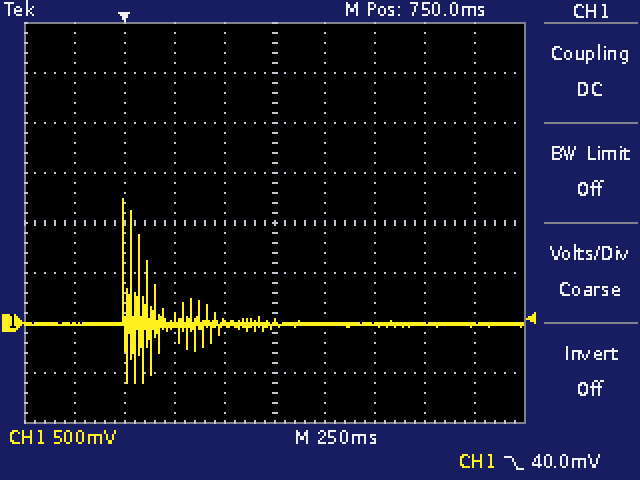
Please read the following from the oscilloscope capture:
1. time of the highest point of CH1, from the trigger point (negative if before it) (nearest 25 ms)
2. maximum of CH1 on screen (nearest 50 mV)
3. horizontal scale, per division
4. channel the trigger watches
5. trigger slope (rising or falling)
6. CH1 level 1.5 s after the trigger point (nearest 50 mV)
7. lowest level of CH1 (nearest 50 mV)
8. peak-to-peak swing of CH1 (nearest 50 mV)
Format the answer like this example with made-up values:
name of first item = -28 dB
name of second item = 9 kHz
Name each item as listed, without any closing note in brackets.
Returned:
time of the highest point of CH1, from the trigger point (negative if before it) = 0 ms
maximum of CH1 on screen = 1.25 V
horizontal scale, per division = 250 ms
channel the trigger watches = CH1
trigger slope = falling
CH1 level 1.5 s after the trigger point = 0 mV
lowest level of CH1 = -600 mV
peak-to-peak swing of CH1 = 1.85 V
